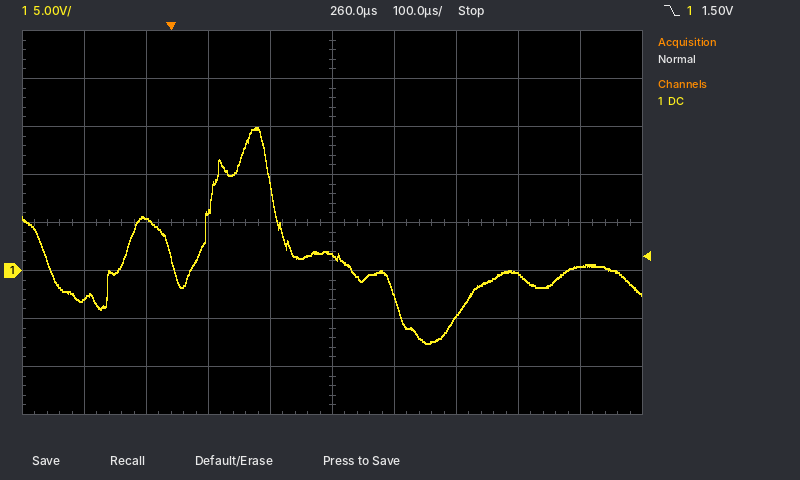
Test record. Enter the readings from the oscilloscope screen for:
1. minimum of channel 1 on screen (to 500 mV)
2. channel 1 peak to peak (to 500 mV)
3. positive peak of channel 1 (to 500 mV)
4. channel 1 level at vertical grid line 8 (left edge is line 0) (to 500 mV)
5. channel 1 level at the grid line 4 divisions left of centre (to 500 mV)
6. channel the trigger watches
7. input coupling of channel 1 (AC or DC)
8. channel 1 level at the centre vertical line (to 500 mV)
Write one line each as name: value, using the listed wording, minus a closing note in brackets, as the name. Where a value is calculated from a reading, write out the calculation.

minimum of channel 1 on screen: -7.5 V
channel 1 peak to peak: 15.0 V − (-7.5 V) = 22.5 V
positive peak of channel 1: 15.0 V
channel 1 level at vertical grid line 8 (left edge is line 0): -500 mV
channel 1 level at the grid line 4 divisions left of centre: -3.0 V
channel the trigger watches: channel 1
input coupling of channel 1: DC
channel 1 level at the centre vertical line: 1.5 V
